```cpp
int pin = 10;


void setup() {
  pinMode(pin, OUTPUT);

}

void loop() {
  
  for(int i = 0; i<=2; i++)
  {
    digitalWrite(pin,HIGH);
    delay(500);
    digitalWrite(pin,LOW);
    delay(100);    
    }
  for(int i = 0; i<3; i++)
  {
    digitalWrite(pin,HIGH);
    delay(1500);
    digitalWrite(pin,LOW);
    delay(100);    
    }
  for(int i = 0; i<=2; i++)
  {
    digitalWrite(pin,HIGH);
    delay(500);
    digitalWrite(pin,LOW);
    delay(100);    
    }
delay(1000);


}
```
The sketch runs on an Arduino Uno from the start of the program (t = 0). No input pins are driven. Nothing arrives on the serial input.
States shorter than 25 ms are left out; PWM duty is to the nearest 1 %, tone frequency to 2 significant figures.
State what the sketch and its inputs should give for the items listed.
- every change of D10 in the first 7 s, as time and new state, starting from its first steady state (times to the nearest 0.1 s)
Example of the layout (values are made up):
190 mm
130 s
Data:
0 s high; 0.5 s low; 0.6 s high; 1.1 s low; 1.2 s high; 1.7 s low; 1.8 s high; 3.3 s low; 3.4 s high; 4.9 s low; 5 s high; 6.5 s low; 6.6 s high
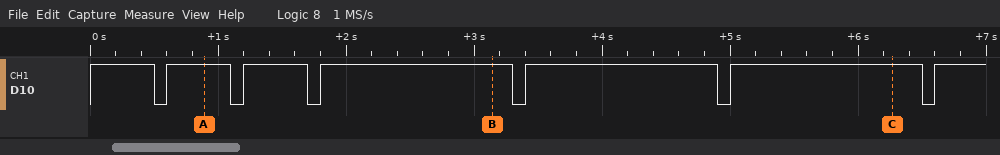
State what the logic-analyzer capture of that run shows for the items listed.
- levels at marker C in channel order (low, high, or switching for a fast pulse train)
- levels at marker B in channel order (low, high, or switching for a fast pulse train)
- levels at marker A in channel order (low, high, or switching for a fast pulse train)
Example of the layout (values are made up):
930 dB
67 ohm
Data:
D10 high
D10 high
D10 high
